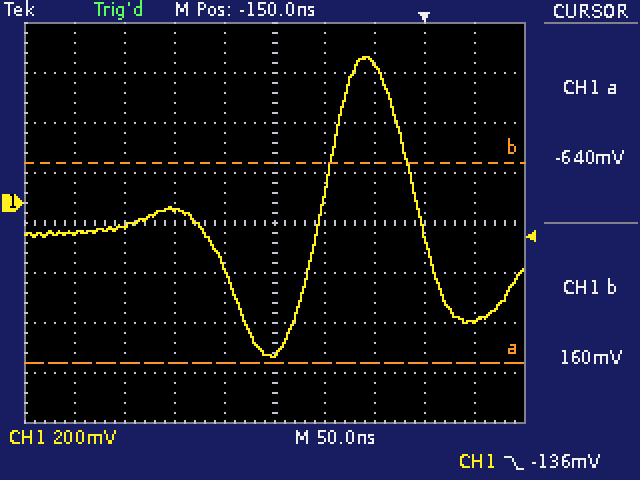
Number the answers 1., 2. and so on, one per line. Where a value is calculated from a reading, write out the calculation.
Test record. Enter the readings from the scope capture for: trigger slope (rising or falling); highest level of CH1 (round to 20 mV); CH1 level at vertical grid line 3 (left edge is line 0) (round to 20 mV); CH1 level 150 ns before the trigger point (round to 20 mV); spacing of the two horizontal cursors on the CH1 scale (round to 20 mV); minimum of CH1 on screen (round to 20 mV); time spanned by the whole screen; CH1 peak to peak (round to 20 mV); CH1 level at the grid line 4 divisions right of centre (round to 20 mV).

1. falling
2. 580 mV
3. -20 mV
4. -600 mV
5. 800 mV
6. -620 mV
7. 500 ns
8. 580 mV − (-620 mV) = 1.20 V
9. -480 mV
